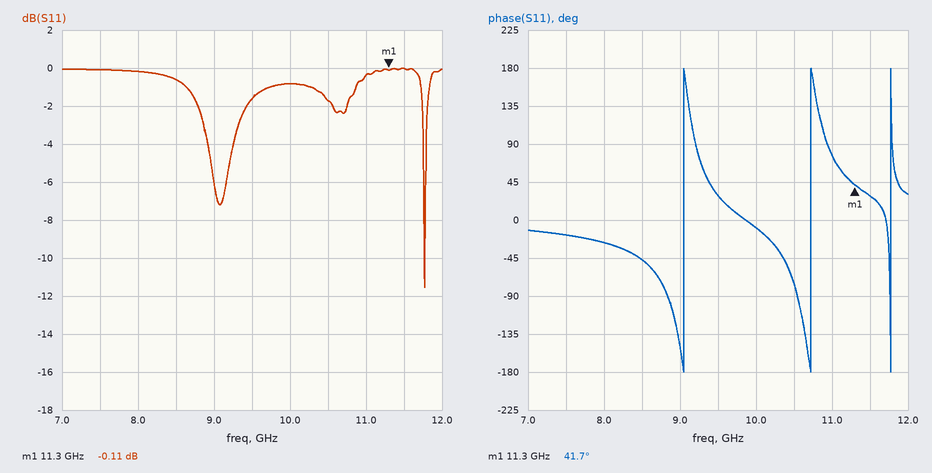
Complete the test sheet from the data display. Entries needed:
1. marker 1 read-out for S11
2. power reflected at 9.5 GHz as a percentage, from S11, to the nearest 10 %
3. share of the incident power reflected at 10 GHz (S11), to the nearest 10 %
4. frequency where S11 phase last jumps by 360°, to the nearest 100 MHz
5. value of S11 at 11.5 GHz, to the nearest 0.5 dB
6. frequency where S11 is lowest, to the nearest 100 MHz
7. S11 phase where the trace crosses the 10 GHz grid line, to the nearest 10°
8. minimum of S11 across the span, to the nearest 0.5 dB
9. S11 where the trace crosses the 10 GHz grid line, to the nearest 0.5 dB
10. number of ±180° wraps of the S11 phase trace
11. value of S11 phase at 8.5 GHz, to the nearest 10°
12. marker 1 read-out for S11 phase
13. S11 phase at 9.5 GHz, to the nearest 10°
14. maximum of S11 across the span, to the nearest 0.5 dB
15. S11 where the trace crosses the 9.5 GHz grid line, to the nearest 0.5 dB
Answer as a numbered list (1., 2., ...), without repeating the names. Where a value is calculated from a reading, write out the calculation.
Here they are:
1. -0.11 dB
2. 10^(-1.5/10) ≈ 70.8 %, so 70 % to the nearest 10 %
3. 10^(-1/10) ≈ 79.4 %, so 80 % to the nearest 10 %
4. 11.8 GHz
5. 0.0 dB
6. 11.8 GHz
7. -10°
8. -11.5 dB
9. -1.0 dB
10. 3
11. -50°
12. 41.7°
13. 30°
14. 0.0 dB
15. -1.5 dB
